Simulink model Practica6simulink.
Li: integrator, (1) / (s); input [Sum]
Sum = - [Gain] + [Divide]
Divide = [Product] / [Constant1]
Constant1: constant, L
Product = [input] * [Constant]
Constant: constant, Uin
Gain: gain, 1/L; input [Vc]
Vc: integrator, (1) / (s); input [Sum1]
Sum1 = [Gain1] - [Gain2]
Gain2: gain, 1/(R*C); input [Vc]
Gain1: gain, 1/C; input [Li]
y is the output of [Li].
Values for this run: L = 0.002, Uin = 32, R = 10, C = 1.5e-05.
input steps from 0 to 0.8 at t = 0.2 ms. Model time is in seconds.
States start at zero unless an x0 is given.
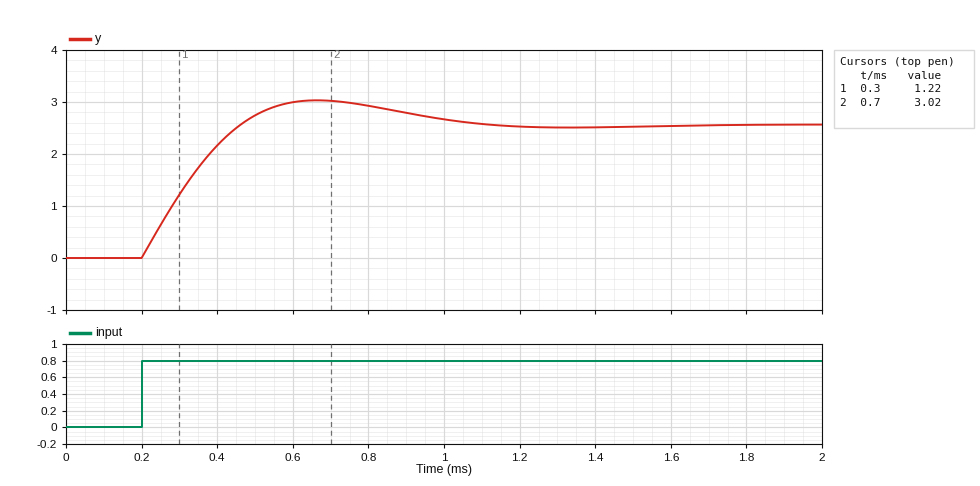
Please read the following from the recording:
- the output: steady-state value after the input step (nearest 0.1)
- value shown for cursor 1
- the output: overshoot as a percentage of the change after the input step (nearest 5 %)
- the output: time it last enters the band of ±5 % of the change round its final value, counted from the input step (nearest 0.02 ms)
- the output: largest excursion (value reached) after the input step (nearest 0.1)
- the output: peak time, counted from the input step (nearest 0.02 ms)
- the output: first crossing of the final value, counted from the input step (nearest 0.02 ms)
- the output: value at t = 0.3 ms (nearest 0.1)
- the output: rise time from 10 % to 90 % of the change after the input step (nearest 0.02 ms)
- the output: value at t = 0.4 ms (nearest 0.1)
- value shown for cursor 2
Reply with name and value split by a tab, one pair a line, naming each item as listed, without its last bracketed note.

the output: steady-state value after the input step	2.6
value shown for cursor 1	1.22
the output: overshoot as a percentage of the change after the input step	20 %
the output: time it last enters the band of ±5 % of the change round its final value, counted from the input step	0.78 ms
the output: largest excursion (value reached) after the input step	3.0
the output: peak time, counted from the input step	0.46 ms
the output: first crossing of the final value, counted from the input step	0.26 ms
the output: value at t = 0.3 ms	1.2
the output: rise time from 10 % to 90 % of the change after the input step	0.20 ms
the output: value at t = 0.4 ms	2.2
value shown for cursor 2	3.02
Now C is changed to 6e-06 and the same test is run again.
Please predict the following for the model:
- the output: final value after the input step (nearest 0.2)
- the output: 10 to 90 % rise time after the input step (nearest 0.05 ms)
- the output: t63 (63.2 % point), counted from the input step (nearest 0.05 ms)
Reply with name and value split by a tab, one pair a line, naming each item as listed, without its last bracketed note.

the output: final value after the input step	2.6
the output: 10 to 90 % rise time after the input step	0.30 ms
the output: t63 (63.2 % point), counted from the input step	0.15 ms
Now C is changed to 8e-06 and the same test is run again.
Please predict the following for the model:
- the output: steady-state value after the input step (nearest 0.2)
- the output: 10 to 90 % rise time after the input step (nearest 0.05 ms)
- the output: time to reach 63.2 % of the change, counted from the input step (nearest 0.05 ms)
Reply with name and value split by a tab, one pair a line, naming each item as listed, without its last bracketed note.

the output: steady-state value after the input step	2.6
the output: 10 to 90 % rise time after the input step	0.25 ms
the output: time to reach 63.2 % of the change, counted from the input step	0.15 ms
